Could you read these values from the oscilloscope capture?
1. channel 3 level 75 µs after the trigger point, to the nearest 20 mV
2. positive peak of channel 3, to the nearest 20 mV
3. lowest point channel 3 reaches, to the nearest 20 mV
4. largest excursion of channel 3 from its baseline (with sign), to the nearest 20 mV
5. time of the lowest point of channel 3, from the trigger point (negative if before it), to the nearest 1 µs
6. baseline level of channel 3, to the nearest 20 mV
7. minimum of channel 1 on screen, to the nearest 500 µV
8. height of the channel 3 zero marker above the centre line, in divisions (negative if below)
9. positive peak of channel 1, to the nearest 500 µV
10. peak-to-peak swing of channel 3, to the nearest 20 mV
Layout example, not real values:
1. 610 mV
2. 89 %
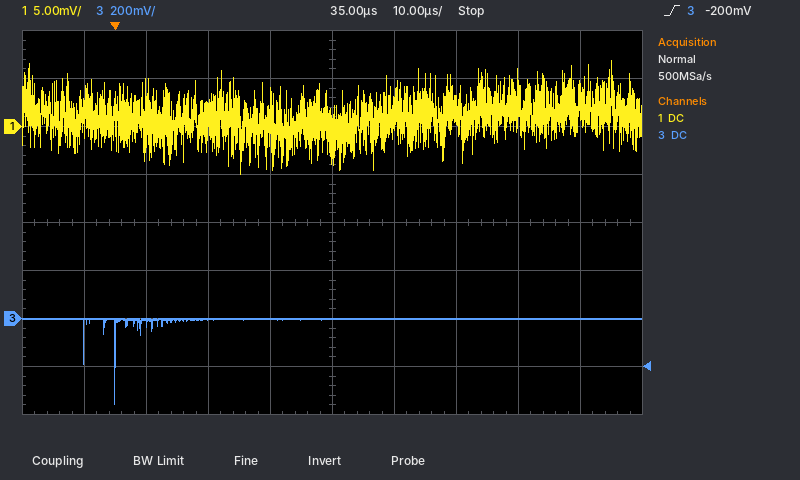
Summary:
1. 0 mV
2. 0 mV
3. -360 mV
4. -360 mV
5. 0 µs
6. 0 mV
7. -5.0 mV
8. -2.0 div
9. 7.0 mV
10. 360 mV
